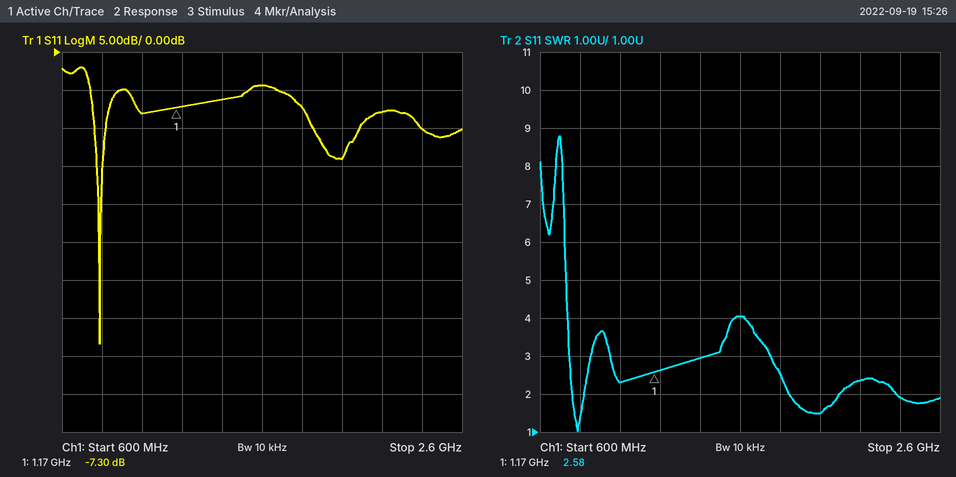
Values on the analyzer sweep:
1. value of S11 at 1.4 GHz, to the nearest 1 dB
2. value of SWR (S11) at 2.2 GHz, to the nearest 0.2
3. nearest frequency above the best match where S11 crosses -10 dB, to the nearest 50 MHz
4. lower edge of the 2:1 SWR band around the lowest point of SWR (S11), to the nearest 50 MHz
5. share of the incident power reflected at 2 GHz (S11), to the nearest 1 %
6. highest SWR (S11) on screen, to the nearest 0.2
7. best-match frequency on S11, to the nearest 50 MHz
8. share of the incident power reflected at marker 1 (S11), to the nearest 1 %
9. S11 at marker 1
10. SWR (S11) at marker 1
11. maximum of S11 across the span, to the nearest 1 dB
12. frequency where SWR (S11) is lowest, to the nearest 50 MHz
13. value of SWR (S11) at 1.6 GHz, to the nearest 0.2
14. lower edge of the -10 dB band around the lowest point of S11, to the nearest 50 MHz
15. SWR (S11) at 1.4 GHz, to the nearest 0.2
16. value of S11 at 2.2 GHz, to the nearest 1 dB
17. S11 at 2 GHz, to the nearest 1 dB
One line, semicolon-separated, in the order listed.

-6 dB; 2.4; 800 MHz; 750 MHz; 4 %; 8.8; 800 MHz; 19 %; -7.30 dB; 2.58; -2 dB; 800 MHz; 4.0; 750 MHz; 3.0; -8 dB; -14 dB
